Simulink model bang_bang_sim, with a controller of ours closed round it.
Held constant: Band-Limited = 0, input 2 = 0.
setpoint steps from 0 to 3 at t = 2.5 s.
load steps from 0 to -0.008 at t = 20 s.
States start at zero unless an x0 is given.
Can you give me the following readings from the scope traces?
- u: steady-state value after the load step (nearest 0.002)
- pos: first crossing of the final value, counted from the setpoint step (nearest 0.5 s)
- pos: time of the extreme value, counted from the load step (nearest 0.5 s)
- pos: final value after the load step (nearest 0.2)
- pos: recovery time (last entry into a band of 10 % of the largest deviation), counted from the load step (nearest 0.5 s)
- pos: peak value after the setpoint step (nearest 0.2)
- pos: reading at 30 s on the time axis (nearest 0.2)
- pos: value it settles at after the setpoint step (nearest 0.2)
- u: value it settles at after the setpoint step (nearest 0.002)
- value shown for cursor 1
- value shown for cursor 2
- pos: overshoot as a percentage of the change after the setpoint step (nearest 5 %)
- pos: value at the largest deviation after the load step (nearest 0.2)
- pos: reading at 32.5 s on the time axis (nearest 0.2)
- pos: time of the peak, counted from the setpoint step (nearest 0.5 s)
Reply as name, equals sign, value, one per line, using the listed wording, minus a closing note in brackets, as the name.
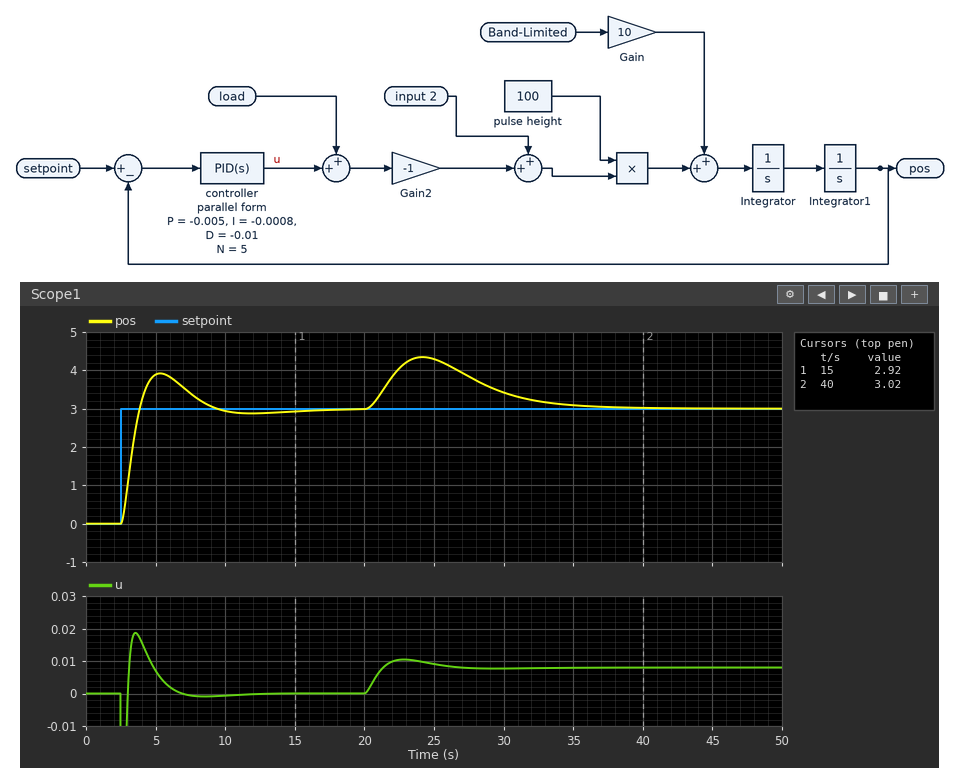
u: steady-state value after the load step = 0.008
pos: first crossing of the final value, counted from the setpoint step = 1.5 s
pos: time of the extreme value, counted from the load step = 4.0 s
pos: final value after the load step = 3.0
pos: recovery time (last entry into a band of 10 % of the largest deviation), counted from the load step = 13.5 s
pos: peak value after the setpoint step = 4.0
pos: reading at 30 s on the time axis = 3.4
pos: value it settles at after the setpoint step = 3.0
u: value it settles at after the setpoint step = 0.000
value shown for cursor 1 = 2.92
value shown for cursor 2 = 3.02
pos: overshoot as a percentage of the change after the setpoint step = 30 %
pos: value at the largest deviation after the load step = 4.4
pos: reading at 32.5 s on the time axis = 3.2
pos: time of the peak, counted from the setpoint step = 3.0 s
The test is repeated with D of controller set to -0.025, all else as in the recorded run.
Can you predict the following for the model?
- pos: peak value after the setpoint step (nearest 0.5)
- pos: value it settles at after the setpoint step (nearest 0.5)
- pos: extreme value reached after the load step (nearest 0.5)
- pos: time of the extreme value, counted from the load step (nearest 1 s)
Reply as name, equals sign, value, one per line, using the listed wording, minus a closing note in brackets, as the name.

pos: peak value after the setpoint step = 3.5
pos: value it settles at after the setpoint step = 3.0
pos: extreme value reached after the load step = 4.0
pos: time of the extreme value, counted from the load step = 7 s
